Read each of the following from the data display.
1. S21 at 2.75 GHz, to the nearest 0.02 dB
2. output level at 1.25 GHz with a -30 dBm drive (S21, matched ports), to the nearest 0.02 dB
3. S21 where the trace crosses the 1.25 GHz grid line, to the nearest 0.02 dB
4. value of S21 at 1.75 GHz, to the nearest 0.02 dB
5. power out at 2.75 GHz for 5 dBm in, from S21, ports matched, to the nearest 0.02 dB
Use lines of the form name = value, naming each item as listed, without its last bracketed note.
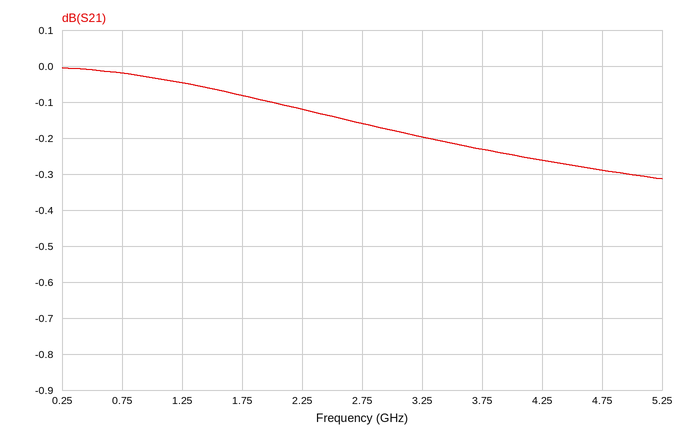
S21 at 2.75 GHz, to the nearest 0.02 dB = -0.16 dB
output level at 1.25 GHz with a -30 dBm drive (S21, matched ports), to the nearest 0.02 dB = -30.04 dBm
S21 where the trace crosses the 1.25 GHz grid line, to the nearest 0.02 dB = -0.04 dB
value of S21 at 1.75 GHz, to the nearest 0.02 dB = -0.08 dB
power out at 2.75 GHz for 5 dBm in, from S21, ports matched, to the nearest 0.02 dB = 4.84 dBm
